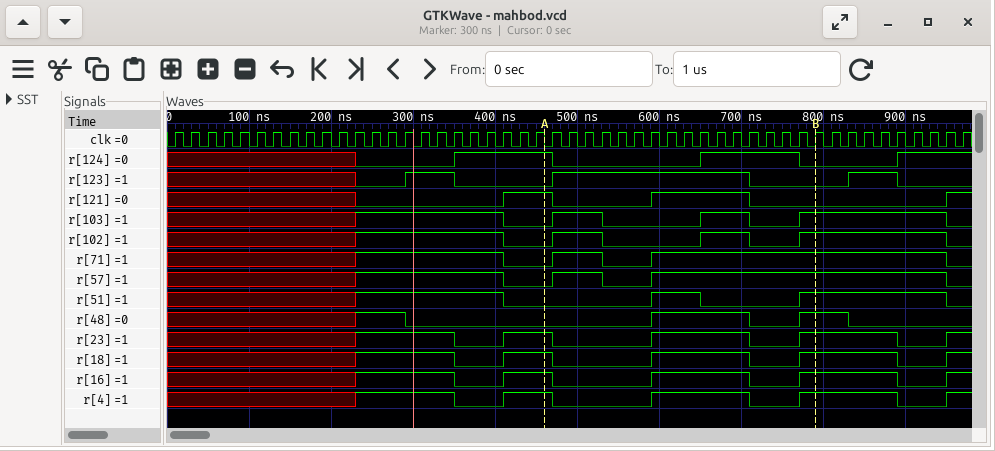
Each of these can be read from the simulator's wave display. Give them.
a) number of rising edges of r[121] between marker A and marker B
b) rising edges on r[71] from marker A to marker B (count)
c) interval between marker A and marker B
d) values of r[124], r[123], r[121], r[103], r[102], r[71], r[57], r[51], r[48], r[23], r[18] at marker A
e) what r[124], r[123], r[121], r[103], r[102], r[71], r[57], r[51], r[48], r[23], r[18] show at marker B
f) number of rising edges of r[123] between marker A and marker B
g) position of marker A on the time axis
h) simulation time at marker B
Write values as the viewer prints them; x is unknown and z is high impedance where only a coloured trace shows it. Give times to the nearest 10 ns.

1
2
330 ns
r[124]=1, r[123]=0, r[121]=1, r[103]=0, r[102]=0, r[71]=0, r[57]=0, r[51]=0, r[48]=0, r[23]=1, r[18]=1
r[124]=0, r[123]=0, r[121]=0, r[103]=1, r[102]=1, r[71]=1, r[57]=1, r[51]=1, r[48]=1, r[23]=1, r[18]=1
1
460 ns
790 ns
